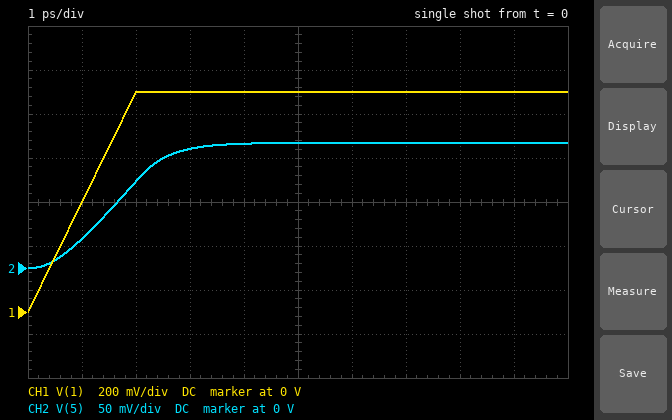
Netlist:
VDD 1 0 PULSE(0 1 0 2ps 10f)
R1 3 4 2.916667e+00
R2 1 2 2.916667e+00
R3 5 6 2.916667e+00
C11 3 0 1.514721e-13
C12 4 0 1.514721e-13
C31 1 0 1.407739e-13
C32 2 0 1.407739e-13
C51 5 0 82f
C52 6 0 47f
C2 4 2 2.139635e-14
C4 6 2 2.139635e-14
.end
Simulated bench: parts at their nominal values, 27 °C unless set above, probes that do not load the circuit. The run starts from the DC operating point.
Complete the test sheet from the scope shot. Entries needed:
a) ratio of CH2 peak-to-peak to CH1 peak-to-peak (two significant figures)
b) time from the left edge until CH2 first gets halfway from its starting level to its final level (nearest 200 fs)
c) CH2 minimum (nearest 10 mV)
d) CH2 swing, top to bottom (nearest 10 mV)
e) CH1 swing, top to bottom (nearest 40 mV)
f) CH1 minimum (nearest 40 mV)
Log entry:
0.14
1.6 ps
0 V
140 mV
1.00 V
0 V
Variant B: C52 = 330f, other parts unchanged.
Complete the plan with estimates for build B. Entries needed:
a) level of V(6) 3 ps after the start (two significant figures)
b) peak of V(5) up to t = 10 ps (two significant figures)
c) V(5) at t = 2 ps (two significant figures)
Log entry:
48 mV
49 mV
32 mV
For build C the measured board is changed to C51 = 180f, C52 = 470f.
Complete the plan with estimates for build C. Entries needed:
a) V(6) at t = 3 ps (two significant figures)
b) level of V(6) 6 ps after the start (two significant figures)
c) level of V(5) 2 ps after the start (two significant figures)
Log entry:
31 mV
32 mV
18 mV
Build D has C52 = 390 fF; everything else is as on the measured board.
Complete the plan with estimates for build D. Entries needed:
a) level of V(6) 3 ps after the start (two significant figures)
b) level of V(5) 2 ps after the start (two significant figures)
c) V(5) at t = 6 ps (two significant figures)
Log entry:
42 mV
28 mV
43 mV
